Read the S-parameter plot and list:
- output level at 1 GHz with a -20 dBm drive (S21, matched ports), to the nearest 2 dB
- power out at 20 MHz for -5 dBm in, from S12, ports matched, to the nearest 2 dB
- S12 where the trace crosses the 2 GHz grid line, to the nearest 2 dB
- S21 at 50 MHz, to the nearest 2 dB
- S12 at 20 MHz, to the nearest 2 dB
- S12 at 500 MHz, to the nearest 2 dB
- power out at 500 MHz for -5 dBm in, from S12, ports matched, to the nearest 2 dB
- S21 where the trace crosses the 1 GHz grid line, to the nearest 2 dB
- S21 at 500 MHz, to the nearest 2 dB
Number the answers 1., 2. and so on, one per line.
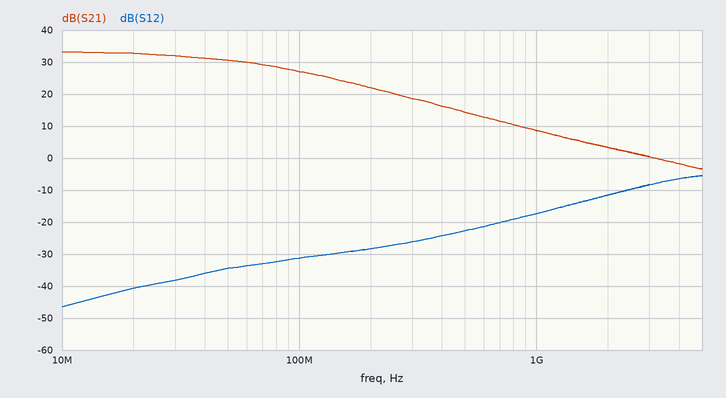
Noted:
1. -12 dBm
2. -46 dBm
3. -12 dB
4. 30 dB
5. -40 dB
6. -22 dB
7. -28 dBm
8. 8 dB
9. 14 dB
